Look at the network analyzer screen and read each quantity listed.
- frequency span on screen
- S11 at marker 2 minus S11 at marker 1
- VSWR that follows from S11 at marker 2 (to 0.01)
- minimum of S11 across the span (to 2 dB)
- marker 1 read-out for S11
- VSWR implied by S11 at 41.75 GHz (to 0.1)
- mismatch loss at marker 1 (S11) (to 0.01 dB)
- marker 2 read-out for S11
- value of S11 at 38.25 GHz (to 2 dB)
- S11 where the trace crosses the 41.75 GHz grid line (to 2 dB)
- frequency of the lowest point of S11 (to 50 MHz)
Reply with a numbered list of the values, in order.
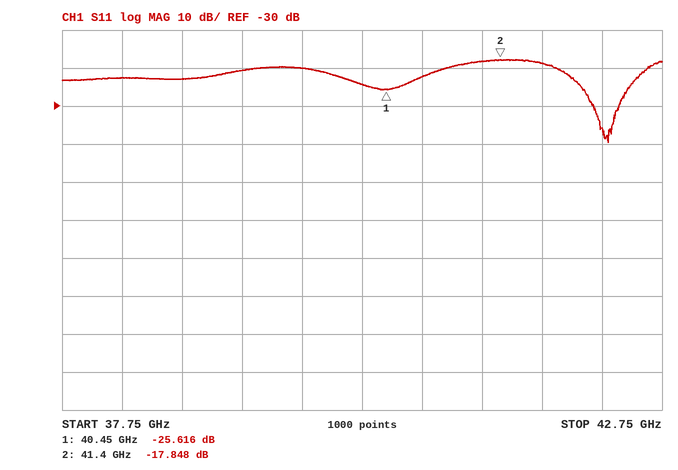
1. 5 GHz
2. 7.768 dB
3. 1.29
4. -40 dB
5. -25.616 dB
6. 1.3
7. 0.01 dB
8. -17.848 dB
9. -22 dB
10. -18 dB
11. 42.30 GHz
